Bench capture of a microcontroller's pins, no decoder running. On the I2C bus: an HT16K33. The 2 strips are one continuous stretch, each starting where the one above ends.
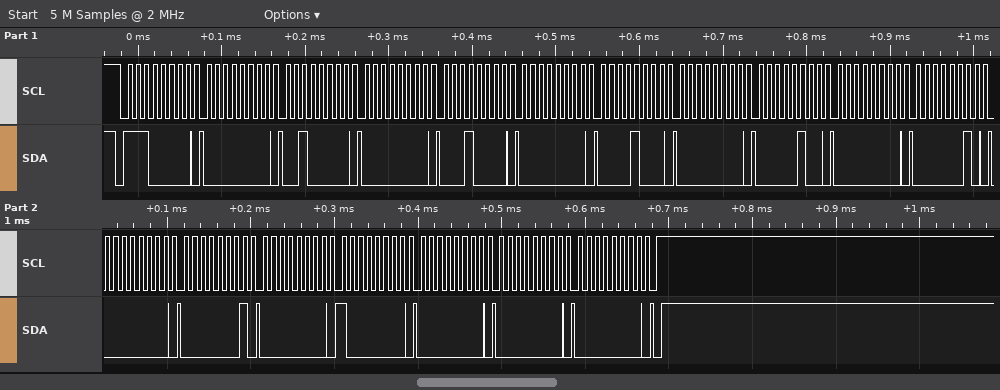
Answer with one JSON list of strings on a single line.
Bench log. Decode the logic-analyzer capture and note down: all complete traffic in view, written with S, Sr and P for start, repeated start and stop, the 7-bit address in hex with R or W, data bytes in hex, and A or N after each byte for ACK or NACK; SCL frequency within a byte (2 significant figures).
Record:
["S 70W A 00 A 20 A 00 A 10 A 00 A 08 A 00 A 04 A 00 A 02 A 00 A 01 A 00 A 80 A 00 A 00 A 00 A P", "100 kHz"]
